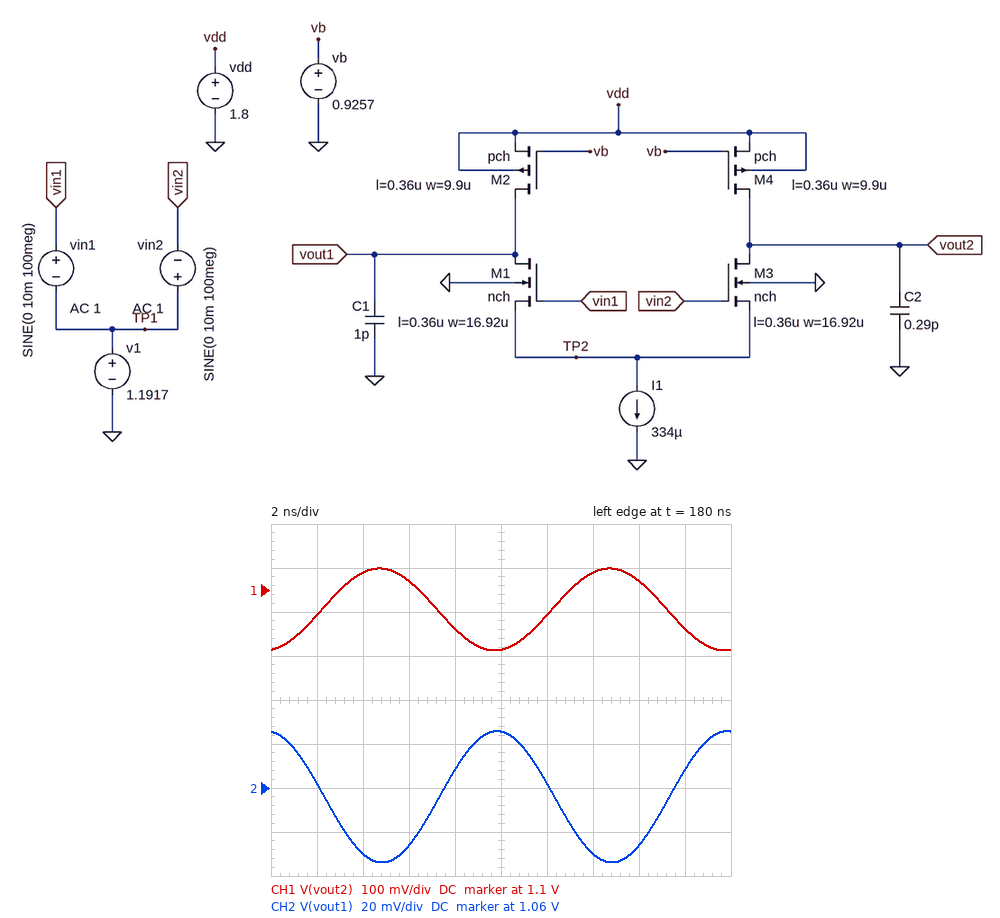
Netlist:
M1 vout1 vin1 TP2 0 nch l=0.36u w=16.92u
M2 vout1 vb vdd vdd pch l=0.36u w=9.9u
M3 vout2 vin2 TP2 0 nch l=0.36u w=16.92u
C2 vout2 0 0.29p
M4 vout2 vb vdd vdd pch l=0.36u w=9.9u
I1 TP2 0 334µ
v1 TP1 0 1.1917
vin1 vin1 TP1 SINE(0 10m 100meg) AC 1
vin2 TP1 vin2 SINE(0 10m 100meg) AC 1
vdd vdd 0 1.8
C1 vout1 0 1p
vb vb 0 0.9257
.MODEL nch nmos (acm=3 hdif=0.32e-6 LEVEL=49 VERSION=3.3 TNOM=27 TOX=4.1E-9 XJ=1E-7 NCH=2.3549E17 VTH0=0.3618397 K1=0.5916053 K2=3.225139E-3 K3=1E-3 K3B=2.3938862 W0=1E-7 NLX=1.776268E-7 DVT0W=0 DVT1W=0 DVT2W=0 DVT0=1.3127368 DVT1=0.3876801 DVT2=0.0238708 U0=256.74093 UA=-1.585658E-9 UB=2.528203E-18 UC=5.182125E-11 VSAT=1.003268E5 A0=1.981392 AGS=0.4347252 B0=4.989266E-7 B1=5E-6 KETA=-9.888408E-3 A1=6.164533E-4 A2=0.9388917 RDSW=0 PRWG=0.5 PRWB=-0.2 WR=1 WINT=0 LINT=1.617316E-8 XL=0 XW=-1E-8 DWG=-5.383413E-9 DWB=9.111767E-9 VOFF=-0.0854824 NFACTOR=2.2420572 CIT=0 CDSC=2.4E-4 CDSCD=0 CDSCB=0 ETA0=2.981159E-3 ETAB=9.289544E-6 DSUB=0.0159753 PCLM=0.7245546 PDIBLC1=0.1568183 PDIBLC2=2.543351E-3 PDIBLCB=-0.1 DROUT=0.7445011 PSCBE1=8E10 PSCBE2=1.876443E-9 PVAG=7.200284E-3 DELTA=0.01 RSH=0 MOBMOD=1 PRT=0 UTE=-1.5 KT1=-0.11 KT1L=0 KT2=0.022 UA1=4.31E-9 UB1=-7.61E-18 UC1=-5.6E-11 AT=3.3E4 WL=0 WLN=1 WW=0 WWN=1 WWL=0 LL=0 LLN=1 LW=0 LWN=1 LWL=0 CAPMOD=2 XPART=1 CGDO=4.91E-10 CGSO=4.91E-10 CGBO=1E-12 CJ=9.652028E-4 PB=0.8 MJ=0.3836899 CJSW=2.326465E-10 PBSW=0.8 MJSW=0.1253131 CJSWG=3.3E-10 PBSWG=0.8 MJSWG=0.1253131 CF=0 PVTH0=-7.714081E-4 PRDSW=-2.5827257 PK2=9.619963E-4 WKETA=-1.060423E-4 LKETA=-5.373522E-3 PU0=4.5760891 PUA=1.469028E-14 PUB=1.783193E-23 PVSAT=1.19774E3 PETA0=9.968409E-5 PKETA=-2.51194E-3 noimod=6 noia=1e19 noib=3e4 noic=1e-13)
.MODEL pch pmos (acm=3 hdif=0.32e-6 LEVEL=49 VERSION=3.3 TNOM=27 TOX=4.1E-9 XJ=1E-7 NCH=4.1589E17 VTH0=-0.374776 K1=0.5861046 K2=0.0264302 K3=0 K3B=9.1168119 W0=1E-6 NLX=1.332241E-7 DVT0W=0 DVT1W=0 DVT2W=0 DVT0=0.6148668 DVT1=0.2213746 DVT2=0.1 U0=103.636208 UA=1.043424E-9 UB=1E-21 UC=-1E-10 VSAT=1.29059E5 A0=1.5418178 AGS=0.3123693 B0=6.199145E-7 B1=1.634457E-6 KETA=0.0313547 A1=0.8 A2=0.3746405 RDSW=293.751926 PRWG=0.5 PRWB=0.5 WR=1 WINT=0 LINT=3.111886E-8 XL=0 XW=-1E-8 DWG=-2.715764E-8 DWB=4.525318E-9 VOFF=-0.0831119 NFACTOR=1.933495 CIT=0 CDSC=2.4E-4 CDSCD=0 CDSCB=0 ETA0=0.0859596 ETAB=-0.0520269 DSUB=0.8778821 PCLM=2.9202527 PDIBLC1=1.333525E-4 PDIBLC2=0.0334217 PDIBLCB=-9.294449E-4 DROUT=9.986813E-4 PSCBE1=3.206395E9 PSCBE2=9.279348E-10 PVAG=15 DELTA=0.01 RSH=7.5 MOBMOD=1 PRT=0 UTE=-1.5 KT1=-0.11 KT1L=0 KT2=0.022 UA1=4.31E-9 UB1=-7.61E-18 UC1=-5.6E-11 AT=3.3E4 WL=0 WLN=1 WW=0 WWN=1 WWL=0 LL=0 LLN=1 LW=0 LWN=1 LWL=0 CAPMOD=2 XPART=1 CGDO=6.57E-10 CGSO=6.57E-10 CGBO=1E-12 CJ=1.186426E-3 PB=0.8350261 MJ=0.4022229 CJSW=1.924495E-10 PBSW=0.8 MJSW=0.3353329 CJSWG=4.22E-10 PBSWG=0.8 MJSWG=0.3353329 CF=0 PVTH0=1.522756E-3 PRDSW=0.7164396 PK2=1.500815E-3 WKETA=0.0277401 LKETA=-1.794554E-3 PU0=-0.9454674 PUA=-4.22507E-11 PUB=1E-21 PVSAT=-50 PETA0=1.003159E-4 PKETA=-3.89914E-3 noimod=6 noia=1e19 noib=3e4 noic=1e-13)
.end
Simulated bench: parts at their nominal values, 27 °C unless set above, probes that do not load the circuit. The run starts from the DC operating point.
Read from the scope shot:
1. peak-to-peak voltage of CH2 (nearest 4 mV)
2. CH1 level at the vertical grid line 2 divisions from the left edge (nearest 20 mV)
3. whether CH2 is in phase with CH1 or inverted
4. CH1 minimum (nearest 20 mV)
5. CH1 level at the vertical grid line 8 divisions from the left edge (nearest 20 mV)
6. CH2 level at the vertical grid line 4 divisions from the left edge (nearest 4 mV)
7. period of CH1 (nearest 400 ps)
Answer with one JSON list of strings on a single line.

["60 mV", "1.14 V", "inverted", "960 mV", "1.12 V", "1.068 V", "10.0 ns"]
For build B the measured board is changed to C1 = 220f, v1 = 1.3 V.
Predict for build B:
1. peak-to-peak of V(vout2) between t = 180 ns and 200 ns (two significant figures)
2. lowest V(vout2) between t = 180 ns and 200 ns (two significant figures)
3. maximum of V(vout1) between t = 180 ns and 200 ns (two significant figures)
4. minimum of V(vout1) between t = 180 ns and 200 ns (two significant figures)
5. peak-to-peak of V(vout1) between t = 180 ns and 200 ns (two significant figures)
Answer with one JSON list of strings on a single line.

["180 mV", "960 mV", "1.2 V", "940 mV", "230 mV"]
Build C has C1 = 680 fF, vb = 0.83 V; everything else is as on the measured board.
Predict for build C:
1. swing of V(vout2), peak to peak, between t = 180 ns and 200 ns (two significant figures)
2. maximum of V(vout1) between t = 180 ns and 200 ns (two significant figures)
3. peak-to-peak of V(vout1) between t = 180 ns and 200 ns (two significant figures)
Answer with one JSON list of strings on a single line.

["71 mV", "1.6 V", "57 mV"]
